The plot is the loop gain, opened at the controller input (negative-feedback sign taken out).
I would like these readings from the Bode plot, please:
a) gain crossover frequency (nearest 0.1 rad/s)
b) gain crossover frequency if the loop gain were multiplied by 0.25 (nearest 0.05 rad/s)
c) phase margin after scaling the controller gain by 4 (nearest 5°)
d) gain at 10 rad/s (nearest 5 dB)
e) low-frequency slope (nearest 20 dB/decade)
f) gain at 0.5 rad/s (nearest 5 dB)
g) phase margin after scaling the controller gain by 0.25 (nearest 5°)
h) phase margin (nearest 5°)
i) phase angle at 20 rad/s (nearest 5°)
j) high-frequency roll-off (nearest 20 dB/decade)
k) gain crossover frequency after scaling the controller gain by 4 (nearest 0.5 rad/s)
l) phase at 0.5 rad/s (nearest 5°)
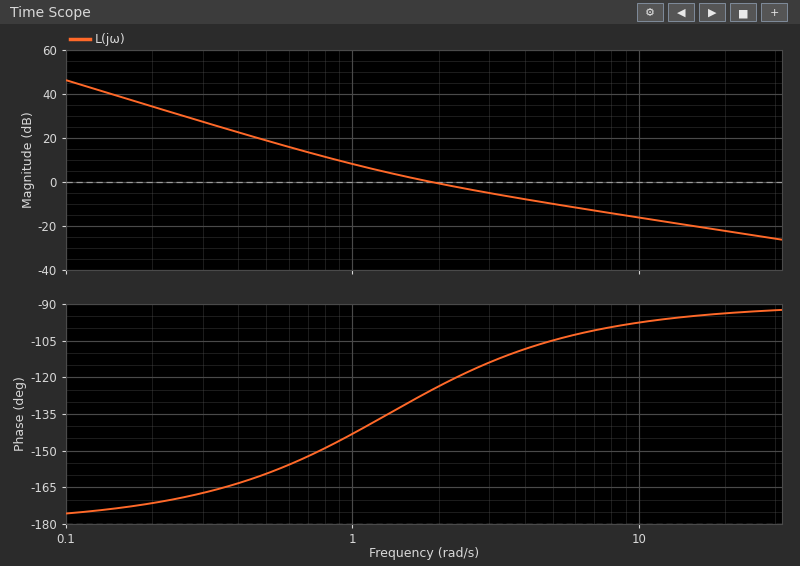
1.9 rad/s
0.75 rad/s
80°
-15 dB
-40 dB/decade
20 dB
30°
55°
-95°
-20 dB/decade
6.5 rad/s
-160°
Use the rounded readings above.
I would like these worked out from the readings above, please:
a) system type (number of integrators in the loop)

2
